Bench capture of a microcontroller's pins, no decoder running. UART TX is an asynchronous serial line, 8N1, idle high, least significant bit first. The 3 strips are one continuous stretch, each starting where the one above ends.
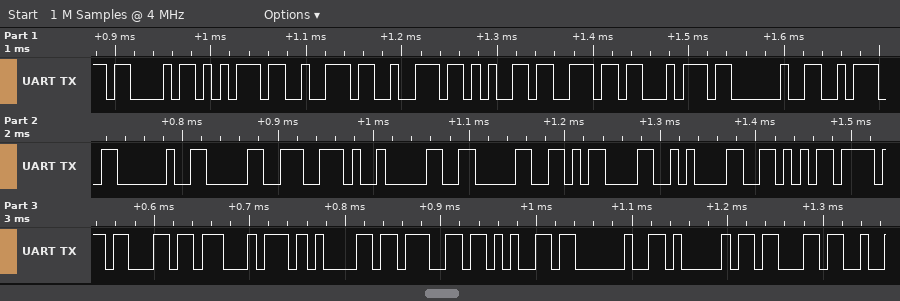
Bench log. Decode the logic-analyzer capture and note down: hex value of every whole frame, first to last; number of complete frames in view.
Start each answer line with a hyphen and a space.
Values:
- 43 75 72 72 65 6E 74 20 3A 20 30 2E 30 30 0D 0A 56 6F 6C 74 61 67 65 20 41 63
- 26
